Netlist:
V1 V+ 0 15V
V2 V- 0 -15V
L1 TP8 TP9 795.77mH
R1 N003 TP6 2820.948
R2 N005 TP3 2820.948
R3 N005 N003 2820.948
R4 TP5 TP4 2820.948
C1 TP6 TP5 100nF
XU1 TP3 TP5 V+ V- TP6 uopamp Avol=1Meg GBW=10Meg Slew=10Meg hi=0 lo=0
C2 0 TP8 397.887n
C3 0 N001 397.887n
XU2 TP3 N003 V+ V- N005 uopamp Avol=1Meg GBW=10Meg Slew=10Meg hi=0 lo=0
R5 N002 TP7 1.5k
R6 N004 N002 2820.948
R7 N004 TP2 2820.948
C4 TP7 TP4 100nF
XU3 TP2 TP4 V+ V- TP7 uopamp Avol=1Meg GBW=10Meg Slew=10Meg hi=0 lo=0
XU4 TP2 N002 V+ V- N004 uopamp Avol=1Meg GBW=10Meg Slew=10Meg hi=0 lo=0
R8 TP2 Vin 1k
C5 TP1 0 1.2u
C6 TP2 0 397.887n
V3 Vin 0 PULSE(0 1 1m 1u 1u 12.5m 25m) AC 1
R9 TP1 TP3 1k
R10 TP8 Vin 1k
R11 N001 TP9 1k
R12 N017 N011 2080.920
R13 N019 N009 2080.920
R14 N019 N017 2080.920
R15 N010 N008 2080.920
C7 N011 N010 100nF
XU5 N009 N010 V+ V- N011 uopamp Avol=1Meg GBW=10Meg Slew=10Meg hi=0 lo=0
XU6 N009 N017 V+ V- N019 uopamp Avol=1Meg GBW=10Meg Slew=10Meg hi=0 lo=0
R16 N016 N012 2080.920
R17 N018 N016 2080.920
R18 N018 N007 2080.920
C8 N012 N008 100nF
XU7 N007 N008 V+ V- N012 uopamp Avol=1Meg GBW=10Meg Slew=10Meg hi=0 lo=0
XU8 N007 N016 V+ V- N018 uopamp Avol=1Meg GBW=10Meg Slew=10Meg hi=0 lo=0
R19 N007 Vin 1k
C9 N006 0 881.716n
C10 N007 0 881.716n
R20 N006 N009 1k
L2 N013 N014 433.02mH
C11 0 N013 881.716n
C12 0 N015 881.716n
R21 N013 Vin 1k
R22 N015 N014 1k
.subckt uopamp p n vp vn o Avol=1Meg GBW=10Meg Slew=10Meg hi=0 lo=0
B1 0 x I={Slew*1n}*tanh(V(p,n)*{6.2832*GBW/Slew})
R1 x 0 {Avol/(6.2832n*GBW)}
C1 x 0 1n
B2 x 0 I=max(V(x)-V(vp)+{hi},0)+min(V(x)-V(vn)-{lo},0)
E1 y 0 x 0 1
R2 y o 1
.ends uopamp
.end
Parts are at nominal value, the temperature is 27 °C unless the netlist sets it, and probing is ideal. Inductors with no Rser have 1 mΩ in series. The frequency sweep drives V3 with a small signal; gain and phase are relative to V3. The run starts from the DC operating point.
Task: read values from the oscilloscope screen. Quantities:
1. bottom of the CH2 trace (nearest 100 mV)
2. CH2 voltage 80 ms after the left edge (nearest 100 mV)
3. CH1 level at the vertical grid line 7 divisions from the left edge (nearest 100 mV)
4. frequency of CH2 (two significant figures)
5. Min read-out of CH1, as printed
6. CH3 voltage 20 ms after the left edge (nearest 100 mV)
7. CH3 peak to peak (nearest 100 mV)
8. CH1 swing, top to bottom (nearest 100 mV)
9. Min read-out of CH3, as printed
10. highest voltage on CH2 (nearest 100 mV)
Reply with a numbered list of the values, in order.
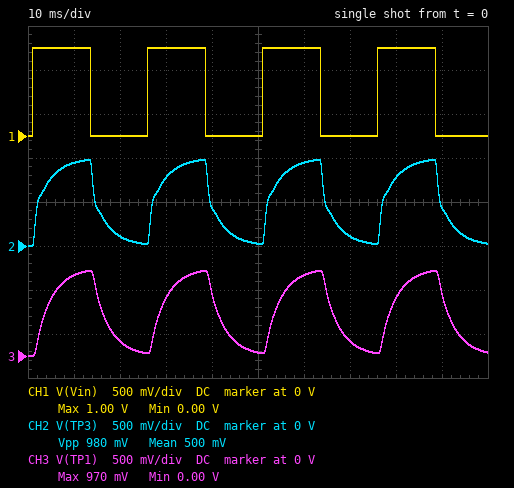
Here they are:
1. 0 V
2. 800 mV
3. 0 V
4. 40 Hz
5. 0.00 V
6. 200 mV
7. 1.0 V
8. 1.0 V
9. 0.00 V
10. 1.0 V
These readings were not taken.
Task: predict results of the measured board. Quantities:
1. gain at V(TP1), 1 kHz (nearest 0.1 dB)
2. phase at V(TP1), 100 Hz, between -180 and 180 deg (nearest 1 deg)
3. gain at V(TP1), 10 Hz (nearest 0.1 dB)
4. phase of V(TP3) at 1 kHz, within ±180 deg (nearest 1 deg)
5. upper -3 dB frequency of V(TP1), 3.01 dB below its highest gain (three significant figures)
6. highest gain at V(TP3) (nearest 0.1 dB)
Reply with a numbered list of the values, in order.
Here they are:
1. -39.0 dB
2. -79 deg
3. -0.2 dB
4. -149 deg
5. 46.1 Hz
6. 0 dB
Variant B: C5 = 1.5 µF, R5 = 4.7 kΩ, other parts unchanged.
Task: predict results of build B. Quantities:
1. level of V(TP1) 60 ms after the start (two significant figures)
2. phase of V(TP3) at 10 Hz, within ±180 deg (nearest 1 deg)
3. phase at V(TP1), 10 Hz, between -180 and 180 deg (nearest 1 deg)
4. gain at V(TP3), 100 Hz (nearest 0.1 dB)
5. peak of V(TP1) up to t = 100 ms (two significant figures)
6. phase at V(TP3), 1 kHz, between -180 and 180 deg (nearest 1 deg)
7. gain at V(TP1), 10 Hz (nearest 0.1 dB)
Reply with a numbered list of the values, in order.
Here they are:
1. 980 mV
2. -5 deg
3. -10 deg
4. -1.7 dB
5. 1.0 V
6. -151 deg
7. -0.1 dB
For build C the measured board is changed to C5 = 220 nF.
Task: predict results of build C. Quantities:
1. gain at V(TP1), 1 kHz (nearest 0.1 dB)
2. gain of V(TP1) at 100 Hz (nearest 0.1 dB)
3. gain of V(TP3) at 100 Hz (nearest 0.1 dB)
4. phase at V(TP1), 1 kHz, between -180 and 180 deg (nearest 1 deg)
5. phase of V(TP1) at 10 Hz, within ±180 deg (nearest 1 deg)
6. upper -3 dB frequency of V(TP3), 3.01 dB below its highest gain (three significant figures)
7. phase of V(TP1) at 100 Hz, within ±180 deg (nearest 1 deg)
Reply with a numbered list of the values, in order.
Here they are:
1. -23.1 dB
2. -0.8 dB
3. -0.7 dB
4. 131 deg
5. -4 deg
6. 385 Hz
7. -35 deg
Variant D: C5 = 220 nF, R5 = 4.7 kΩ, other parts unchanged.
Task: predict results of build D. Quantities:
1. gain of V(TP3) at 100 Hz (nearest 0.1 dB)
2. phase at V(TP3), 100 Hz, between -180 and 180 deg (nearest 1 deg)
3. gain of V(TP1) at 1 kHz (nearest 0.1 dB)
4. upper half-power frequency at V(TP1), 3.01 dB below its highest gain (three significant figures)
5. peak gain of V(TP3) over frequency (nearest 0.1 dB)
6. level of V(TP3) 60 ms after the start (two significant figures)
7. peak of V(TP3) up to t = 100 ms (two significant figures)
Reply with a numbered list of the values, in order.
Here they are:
1. 0 dB
2. -19 deg
3. -23.9 dB
4. 467 Hz
5. 1.4 dB
6. 1.0 V
7. 1.2 V
